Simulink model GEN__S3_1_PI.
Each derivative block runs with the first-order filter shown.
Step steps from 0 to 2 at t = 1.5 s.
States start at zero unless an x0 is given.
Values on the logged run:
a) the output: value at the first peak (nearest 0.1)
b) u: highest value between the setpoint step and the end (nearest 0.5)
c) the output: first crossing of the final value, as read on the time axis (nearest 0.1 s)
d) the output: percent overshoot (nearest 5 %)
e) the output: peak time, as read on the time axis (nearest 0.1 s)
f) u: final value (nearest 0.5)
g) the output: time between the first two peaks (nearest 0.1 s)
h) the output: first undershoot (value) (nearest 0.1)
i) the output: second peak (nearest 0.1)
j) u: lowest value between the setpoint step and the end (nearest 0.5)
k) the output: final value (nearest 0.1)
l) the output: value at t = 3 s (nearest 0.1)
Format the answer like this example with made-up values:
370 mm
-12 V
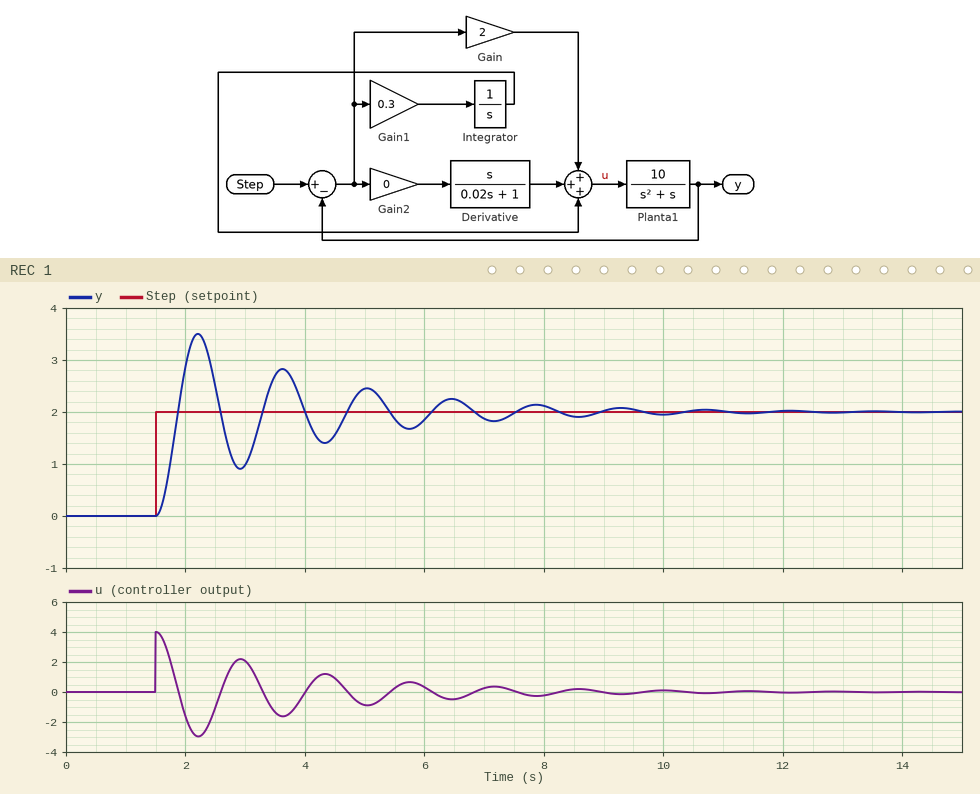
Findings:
3.5
4.0
1.9 s
75 %
2.2 s
0.0
1.4 s
0.9
2.8
-3.0
2.0
1.0
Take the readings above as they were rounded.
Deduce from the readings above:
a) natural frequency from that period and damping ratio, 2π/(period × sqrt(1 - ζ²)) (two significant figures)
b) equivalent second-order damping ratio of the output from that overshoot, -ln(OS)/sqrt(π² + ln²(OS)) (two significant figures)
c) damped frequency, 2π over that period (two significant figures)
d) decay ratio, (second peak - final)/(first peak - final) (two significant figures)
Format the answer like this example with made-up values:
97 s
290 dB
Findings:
4.5 rad/s
0.091
4.5 rad/s
0.53
